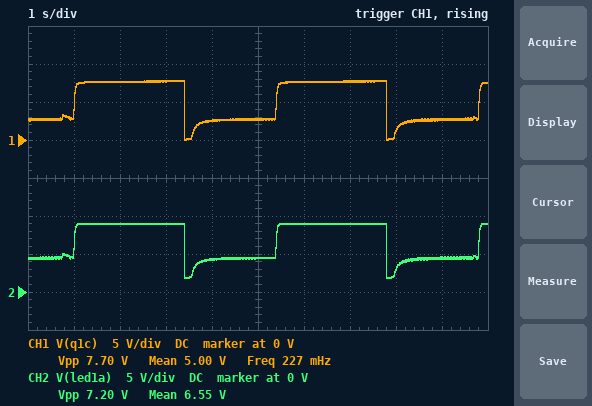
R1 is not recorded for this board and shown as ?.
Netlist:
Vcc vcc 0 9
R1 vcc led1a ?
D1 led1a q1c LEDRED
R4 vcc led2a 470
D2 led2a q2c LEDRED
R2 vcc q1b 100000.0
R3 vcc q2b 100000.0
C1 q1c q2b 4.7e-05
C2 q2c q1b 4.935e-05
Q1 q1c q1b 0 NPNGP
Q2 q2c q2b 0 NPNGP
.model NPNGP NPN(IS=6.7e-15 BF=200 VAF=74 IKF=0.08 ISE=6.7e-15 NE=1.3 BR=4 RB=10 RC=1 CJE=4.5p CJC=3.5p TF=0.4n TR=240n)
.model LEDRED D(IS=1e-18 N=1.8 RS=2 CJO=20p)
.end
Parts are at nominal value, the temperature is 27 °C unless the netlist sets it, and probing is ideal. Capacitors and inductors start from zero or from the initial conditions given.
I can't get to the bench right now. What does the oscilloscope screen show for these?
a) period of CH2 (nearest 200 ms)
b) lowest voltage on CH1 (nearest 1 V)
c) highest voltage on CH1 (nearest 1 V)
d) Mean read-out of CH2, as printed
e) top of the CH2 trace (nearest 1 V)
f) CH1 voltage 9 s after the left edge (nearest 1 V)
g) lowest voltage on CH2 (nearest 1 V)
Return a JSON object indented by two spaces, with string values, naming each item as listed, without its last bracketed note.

{
  "period of CH2": "4.4 s",
  "lowest voltage on CH1": "0 V",
  "highest voltage on CH1": "8 V",
  "Mean read-out of CH2, as printed": "6.55 V",
  "top of the CH2 trace": "9 V",
  "CH1 voltage 9 s after the left edge": "3 V",
  "lowest voltage on CH2": "2 V"
}
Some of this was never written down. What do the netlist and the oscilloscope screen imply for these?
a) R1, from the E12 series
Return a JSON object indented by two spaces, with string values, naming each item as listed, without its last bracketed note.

{
  "R1, from the E12 series": "390 Ω"
}
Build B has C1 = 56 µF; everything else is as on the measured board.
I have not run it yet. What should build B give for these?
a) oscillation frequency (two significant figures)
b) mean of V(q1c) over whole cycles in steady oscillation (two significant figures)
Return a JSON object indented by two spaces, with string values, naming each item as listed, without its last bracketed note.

{
  "oscillation frequency": "210 mHz",
  "mean of V(q1c) over whole cycles in steady oscillation": "5.0 V"
}
